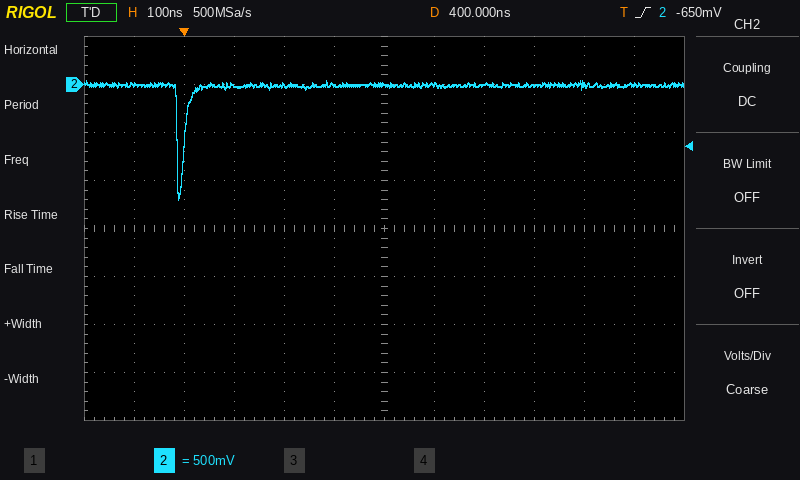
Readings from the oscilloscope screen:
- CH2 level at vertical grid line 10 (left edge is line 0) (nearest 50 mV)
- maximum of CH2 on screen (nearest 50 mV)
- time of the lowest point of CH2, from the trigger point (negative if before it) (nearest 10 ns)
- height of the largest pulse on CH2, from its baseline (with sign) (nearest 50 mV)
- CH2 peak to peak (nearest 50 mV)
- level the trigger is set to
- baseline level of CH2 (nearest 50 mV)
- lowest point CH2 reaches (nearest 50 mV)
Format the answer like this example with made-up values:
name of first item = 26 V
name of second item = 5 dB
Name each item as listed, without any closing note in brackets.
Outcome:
CH2 level at vertical grid line 10 (left edge is line 0) = 0 mV
maximum of CH2 on screen = 50 mV
time of the lowest point of CH2, from the trigger point (negative if before it) = -10 ns
height of the largest pulse on CH2, from its baseline (with sign) = -1.20 V
CH2 peak to peak = 1.25 V
level the trigger is set to = -650 mV
baseline level of CH2 = 0 mV
lowest point CH2 reaches = -1.20 V
